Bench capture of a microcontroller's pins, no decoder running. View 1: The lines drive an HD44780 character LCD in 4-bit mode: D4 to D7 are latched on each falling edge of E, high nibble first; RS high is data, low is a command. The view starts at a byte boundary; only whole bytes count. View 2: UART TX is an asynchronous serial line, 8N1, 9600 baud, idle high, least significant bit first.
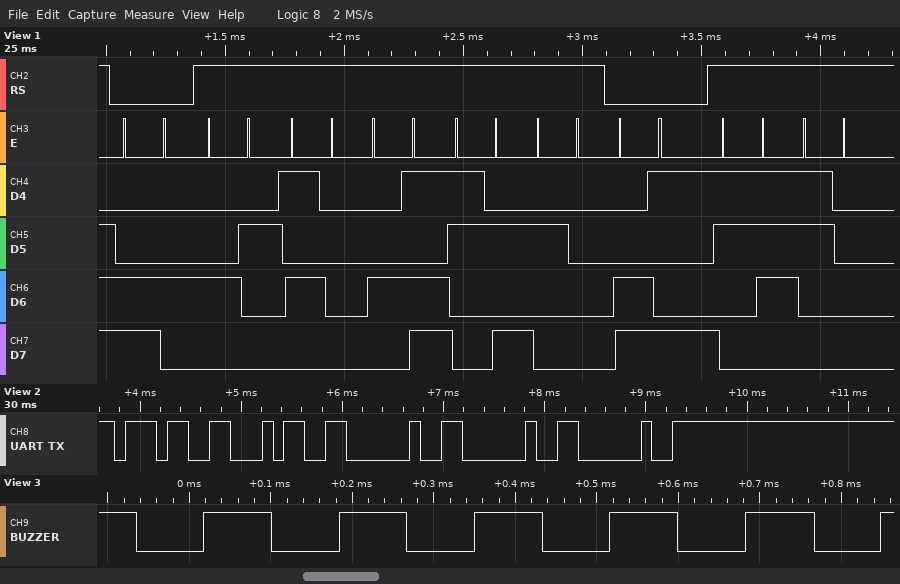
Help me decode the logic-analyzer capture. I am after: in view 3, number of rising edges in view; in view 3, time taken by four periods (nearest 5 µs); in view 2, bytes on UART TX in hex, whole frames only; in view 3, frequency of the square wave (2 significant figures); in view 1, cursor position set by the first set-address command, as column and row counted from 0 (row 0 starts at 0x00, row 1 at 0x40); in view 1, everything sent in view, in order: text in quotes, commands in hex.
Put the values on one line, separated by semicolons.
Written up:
6; 665 µs; 37 34 20 20 20; 6.0 kHz; column 4, row 1; 0xC4 "BPM: " 0xC9 "70"
